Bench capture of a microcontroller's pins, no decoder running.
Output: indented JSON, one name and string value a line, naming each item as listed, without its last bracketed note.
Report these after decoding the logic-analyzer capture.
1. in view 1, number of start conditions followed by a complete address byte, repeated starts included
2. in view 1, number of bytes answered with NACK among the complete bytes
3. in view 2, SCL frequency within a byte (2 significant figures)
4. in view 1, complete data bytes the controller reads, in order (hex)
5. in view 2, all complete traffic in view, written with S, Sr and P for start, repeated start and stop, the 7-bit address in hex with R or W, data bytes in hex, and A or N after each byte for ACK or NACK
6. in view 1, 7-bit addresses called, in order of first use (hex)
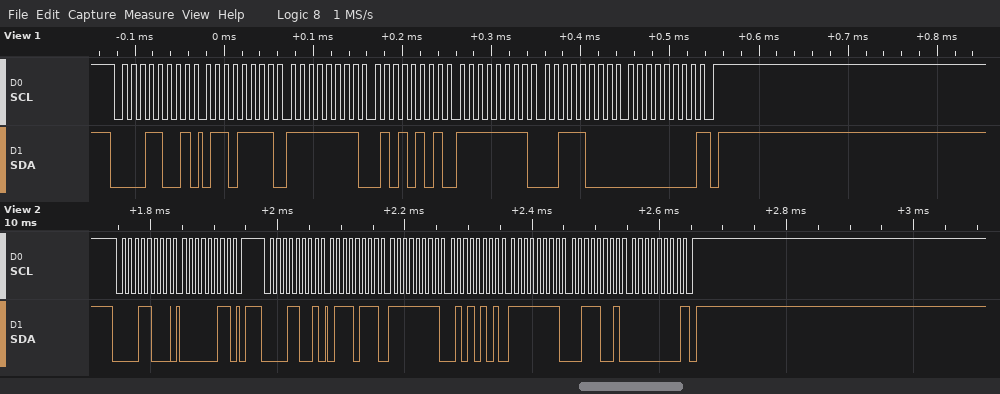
{
  "in view 1, number of start conditions followed by a complete address byte, repeated starts included": "1",
  "in view 1, number of bytes answered with NACK among the complete bytes": "1",
  "in view 2, SCL frequency within a byte": "100 kHz",
  "in view 1, complete data bytes the controller reads, in order": "6F FF 55 FF 38 00",
  "in view 2, all complete traffic in view, written with S, Sr and P for start, repeated start and stop, the 7-bit address in hex with R or W, data bytes in hex, and A or N after each byte for ACK or NACK": "S 0CW A 03 A P S 0CR A 77 A FF A 55 A FF A 39 A 00 N P",
  "in view 1, 7-bit addresses called, in order of first use": "0x0C"
}
